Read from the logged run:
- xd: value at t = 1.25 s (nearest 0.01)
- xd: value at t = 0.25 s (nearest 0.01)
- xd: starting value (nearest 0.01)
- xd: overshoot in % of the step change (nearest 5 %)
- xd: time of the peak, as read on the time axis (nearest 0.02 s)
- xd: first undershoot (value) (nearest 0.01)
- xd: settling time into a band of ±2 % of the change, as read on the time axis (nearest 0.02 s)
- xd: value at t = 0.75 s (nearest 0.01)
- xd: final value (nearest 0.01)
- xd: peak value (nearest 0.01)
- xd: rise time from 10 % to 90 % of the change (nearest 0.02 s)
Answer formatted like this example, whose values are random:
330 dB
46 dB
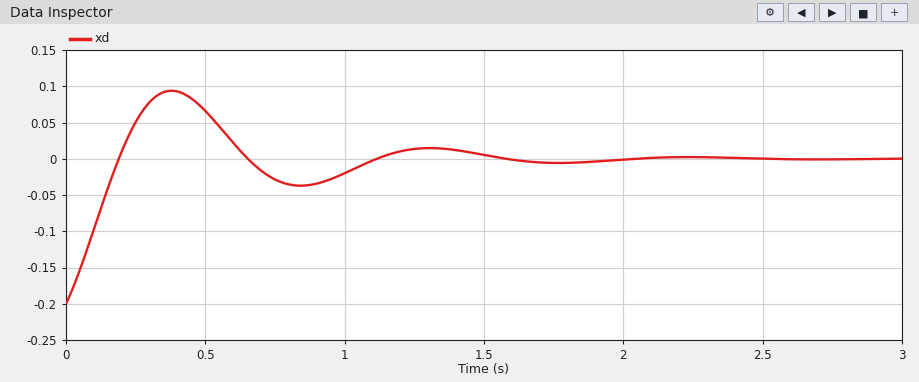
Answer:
0.01
0.05
-0.20
45 %
0.38 s
-0.04
1.90 s
-0.03
0.00
0.09
0.14 s
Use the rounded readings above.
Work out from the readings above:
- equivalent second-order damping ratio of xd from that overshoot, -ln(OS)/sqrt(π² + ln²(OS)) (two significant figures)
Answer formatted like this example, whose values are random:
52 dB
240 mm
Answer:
0.25
